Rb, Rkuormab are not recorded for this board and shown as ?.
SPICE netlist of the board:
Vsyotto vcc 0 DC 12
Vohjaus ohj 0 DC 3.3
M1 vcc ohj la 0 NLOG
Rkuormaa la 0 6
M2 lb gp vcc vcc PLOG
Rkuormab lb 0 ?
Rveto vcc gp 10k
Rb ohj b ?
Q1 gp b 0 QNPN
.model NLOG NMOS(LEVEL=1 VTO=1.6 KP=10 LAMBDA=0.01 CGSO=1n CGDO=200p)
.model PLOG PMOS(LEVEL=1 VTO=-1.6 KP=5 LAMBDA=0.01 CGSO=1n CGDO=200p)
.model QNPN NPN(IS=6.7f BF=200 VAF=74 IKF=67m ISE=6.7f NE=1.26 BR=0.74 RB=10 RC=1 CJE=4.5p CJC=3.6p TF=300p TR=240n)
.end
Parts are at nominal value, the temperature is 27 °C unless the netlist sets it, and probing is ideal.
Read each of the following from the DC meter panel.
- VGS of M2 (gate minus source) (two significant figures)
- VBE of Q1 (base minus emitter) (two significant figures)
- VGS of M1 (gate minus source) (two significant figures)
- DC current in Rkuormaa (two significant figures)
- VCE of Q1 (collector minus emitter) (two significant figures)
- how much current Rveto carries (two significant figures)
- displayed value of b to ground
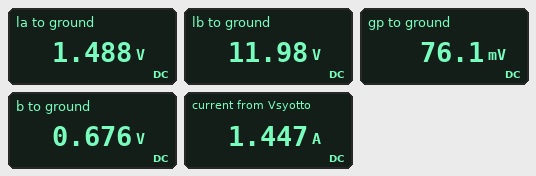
-12 V
680 mV
1.8 V
250 mA
76 mV
1.2 mA
0.676 V
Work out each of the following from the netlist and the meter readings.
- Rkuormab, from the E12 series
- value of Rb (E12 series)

10 Ω
22 kΩ
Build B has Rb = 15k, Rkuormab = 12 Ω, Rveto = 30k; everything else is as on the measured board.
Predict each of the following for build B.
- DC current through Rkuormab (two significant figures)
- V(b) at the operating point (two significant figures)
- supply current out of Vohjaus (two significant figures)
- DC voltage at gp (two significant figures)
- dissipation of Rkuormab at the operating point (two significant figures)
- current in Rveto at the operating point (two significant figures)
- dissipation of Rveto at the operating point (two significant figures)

1.0 A
660 mV
180 µA
45 mV
12 W
400 µA
4.8 mW
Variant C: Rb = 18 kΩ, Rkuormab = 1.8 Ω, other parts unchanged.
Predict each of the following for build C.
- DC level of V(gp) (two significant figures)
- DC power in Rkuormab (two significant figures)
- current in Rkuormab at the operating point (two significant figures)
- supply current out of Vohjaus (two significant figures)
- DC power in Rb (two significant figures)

71 mV
78 W
6.6 A
150 µA
380 µW
